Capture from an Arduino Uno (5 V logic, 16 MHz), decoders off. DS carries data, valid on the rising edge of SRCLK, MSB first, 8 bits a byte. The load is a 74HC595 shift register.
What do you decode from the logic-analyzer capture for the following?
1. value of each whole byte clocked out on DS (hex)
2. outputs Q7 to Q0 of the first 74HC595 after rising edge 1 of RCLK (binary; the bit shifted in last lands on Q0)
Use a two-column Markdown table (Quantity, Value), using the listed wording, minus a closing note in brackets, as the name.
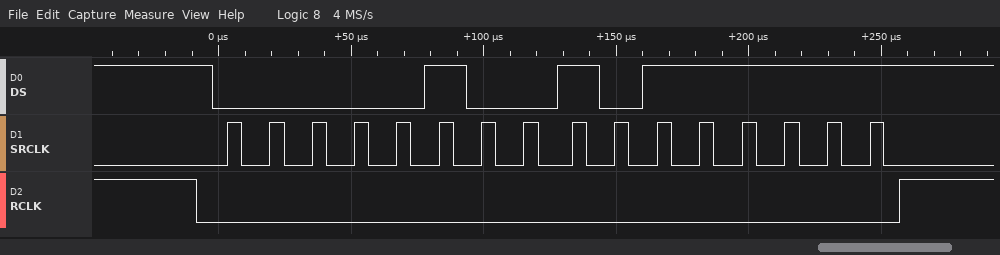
| Quantity | Value |
|---|---|
| value of each whole byte clocked out on DS | 04 BF |
| outputs Q7 to Q0 of the first 74HC595 after rising edge 1 of RCLK | 10111111 |
